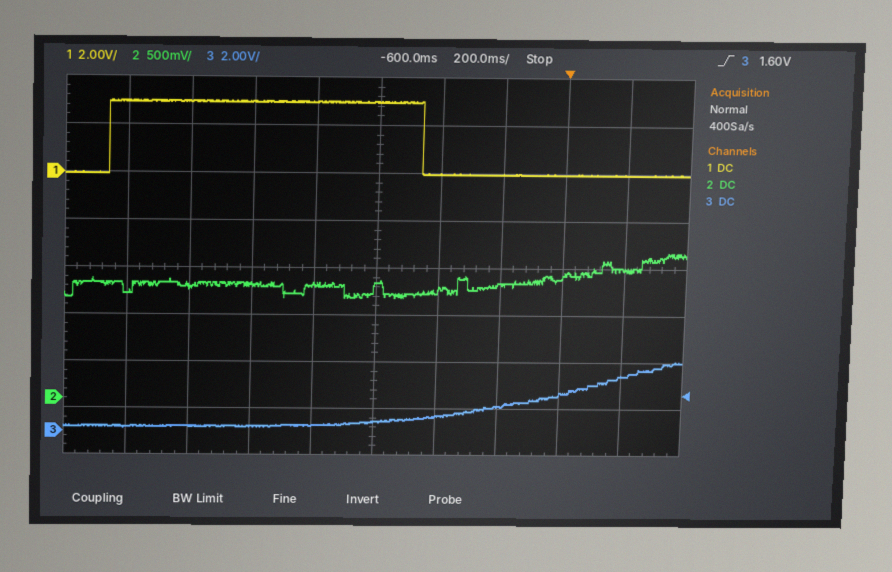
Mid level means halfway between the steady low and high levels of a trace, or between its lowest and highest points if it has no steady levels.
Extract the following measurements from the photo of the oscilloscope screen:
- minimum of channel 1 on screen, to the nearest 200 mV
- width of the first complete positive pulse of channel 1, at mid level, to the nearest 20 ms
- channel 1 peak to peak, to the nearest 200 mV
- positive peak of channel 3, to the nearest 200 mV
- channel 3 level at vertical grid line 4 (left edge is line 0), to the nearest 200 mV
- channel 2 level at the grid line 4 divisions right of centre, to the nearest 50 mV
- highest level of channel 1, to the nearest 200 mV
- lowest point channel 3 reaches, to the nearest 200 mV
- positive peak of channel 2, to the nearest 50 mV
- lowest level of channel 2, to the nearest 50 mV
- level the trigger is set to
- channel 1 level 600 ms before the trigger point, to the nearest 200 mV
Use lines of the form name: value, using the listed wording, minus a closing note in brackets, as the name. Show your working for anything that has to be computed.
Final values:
minimum of channel 1 on screen, to the nearest 200 mV: 0.0 V
width of the first complete positive pulse of channel 1, at mid level, to the nearest 20 ms: 1.00 s
channel 1 peak to peak, to the nearest 200 mV: 3.0 V − (0.0 V) = 3.0 V
positive peak of channel 3, to the nearest 200 mV: 3.0 V
channel 3 level at vertical grid line 4 (left edge is line 0), to the nearest 200 mV: 200 mV
channel 2 level at the grid line 4 divisions right of centre, to the nearest 50 mV: 1.40 V
highest level of channel 1, to the nearest 200 mV: 3.0 V
lowest point channel 3 reaches, to the nearest 200 mV: 200 mV
positive peak of channel 2, to the nearest 50 mV: 1.55 V
lowest level of channel 2, to the nearest 50 mV: 1.10 V
level the trigger is set to: 1.60 V
channel 1 level 600 ms before the trigger point, to the nearest 200 mV: 3.0 V
